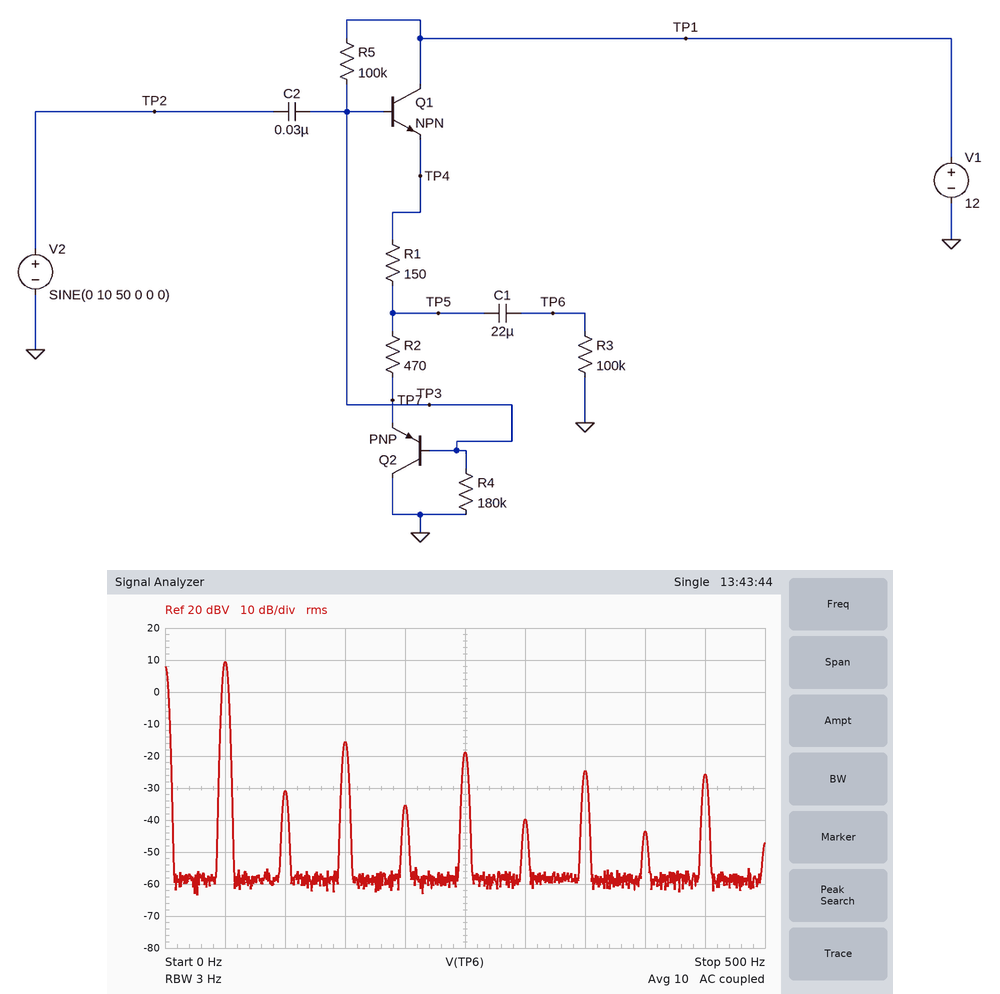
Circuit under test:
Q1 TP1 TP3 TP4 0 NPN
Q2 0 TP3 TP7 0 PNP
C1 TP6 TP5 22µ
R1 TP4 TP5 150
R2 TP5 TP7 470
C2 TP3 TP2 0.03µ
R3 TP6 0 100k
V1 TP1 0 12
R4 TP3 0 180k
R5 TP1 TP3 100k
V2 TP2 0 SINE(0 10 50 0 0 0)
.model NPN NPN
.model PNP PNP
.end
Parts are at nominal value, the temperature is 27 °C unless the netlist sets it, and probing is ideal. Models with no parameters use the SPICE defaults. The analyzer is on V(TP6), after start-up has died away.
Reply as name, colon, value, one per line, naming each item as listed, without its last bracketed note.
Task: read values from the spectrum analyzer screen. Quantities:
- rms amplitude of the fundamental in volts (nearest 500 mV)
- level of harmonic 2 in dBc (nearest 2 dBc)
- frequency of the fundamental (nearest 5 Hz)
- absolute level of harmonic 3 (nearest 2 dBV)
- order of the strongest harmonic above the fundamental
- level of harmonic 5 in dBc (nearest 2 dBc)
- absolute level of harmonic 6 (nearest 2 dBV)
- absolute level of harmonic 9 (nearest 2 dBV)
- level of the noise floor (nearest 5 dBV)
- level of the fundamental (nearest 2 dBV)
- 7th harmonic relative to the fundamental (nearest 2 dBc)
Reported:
rms amplitude of the fundamental in volts: 3.0 V
level of harmonic 2 in dBc: -40 dBc
frequency of the fundamental: 50 Hz
absolute level of harmonic 3: -16 dBV
order of the strongest harmonic above the fundamental: 3
level of harmonic 5 in dBc: -28 dBc
absolute level of harmonic 6: -40 dBV
absolute level of harmonic 9: -26 dBV
level of the noise floor: -60 dBV
level of the fundamental: 10 dBV
7th harmonic relative to the fundamental: -34 dBc
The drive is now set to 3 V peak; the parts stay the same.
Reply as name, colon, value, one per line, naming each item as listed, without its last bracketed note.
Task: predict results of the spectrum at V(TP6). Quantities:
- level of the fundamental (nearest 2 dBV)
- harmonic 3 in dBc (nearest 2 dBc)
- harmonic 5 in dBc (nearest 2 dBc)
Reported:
level of the fundamental: -6 dBV
harmonic 3 in dBc: -12 dBc
harmonic 5 in dBc: -22 dBc
